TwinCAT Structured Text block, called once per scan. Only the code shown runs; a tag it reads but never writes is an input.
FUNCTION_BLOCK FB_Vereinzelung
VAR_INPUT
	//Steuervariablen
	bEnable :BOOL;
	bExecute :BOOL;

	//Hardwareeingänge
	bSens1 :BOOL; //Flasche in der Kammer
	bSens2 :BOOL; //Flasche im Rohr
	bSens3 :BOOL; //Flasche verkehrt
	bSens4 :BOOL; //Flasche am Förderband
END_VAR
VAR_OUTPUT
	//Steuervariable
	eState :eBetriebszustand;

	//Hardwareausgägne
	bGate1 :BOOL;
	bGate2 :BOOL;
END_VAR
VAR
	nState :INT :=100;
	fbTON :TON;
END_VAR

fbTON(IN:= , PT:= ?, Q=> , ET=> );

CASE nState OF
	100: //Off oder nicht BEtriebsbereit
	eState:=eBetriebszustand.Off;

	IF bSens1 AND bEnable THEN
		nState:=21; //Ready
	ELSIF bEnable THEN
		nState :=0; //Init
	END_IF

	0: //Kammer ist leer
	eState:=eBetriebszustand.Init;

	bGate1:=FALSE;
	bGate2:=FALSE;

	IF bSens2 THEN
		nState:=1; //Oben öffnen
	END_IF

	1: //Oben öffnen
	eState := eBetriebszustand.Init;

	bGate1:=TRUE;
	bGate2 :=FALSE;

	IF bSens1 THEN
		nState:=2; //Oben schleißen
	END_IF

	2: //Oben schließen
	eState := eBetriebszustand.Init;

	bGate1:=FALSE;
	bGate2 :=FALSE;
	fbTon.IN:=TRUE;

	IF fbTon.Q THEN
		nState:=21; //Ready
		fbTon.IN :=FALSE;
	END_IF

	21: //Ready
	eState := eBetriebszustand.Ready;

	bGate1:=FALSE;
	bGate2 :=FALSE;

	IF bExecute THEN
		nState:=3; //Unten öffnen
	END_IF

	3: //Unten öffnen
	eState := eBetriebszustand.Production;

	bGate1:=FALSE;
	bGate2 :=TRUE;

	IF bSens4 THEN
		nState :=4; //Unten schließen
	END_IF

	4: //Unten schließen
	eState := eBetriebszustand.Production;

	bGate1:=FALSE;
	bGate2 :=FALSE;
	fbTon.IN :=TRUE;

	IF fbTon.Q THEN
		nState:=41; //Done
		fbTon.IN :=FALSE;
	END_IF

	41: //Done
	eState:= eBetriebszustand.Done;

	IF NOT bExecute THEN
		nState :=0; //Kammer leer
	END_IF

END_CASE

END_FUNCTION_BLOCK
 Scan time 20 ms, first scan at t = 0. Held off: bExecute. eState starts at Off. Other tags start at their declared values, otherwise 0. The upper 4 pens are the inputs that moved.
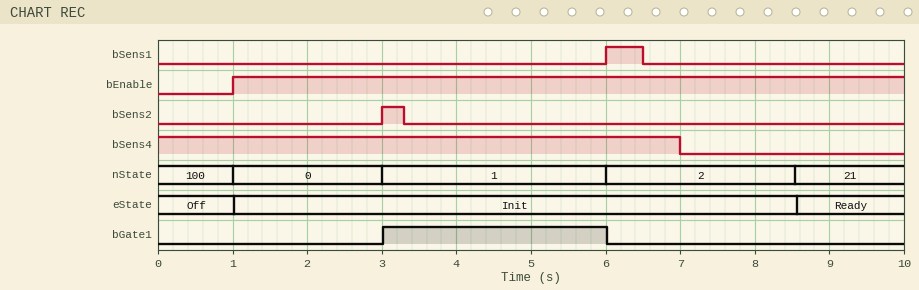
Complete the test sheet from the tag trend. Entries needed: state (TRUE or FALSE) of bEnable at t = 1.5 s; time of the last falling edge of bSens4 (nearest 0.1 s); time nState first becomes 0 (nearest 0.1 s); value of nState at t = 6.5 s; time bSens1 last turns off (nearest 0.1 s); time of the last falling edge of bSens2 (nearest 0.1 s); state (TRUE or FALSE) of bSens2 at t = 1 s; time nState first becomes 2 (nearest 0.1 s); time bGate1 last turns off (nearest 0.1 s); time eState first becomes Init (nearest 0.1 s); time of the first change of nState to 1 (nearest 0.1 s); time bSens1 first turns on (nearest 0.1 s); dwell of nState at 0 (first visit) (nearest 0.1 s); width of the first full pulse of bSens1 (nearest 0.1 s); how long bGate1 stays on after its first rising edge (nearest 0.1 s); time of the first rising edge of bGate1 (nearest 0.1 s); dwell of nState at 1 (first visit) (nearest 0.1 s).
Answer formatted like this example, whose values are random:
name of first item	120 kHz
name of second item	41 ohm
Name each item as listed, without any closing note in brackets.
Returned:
state (TRUE or FALSE) of bEnable at t = 1.5 s	TRUE
time of the last falling edge of bSens4	7.0 s
time nState first becomes 0	1.0 s
value of nState at t = 6.5 s	2
time bSens1 last turns off	6.5 s
time of the last falling edge of bSens2	3.3 s
state (TRUE or FALSE) of bSens2 at t = 1 s	FALSE
time nState first becomes 2	6.0 s
time bGate1 last turns off	6.0 s
time eState first becomes Init	1.0 s
time of the first change of nState to 1	3.0 s
time bSens1 first turns on	6.0 s
dwell of nState at 0 (first visit)	2.0 s
width of the first full pulse of bSens1	0.5 s
how long bGate1 stays on after its first rising edge	3.0 s
time of the first rising edge of bGate1	3.0 s
dwell of nState at 1 (first visit)	3.0 s
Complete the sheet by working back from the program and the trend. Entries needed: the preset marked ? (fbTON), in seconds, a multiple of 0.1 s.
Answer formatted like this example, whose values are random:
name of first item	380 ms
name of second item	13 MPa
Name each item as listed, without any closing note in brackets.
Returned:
the preset marked ? (fbTON), in seconds, a multiple of 0.1 s	2.5 s
